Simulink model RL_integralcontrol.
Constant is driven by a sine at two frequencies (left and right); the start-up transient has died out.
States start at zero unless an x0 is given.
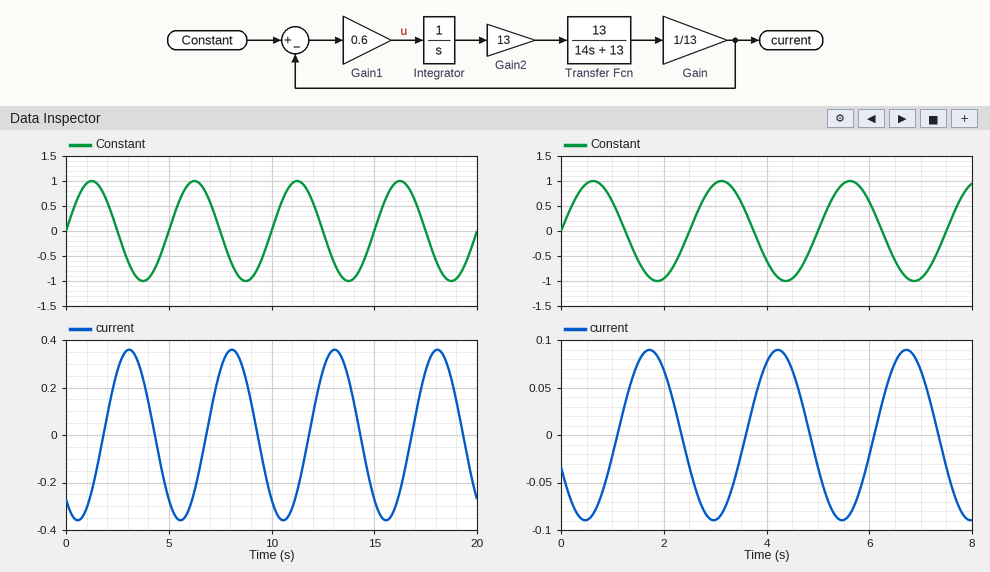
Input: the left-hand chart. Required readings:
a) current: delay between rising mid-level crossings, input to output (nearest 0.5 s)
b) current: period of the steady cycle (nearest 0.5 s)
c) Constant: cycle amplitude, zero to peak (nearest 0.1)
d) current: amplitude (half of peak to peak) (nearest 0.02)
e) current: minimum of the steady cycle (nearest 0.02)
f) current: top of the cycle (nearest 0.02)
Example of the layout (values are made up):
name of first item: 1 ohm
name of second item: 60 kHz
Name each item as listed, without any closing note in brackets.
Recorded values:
current: delay between rising mid-level crossings, input to output: 2.0 s
current: period of the steady cycle: 5.0 s
Constant: cycle amplitude, zero to peak: 1.0
current: amplitude (half of peak to peak): 0.36
current: minimum of the steady cycle: -0.36
current: top of the cycle: 0.36
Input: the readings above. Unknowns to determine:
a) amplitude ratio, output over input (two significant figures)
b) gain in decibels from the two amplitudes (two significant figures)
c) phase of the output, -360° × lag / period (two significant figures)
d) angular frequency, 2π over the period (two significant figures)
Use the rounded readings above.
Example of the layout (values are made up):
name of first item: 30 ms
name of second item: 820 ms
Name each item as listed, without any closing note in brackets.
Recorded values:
amplitude ratio, output over input: 0.36
gain in decibels from the two amplitudes: -8.9 dB
phase of the output, -360° × lag / period: -140°
angular frequency, 2π over the period: 1.3 rad/s
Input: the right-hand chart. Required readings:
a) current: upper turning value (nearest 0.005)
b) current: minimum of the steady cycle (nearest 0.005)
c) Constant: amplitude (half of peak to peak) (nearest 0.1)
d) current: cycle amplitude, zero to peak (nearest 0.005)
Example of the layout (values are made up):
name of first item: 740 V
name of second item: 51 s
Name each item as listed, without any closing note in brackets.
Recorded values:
current: upper turning value: 0.090
current: minimum of the steady cycle: -0.090
Constant: amplitude (half of peak to peak): 1.0
current: cycle amplitude, zero to peak: 0.090
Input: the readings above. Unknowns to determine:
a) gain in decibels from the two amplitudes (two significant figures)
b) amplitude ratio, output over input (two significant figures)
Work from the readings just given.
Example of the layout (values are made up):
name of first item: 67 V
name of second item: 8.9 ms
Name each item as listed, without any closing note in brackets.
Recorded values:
gain in decibels from the two amplitudes: -21 dB
amplitude ratio, output over input: 0.090
